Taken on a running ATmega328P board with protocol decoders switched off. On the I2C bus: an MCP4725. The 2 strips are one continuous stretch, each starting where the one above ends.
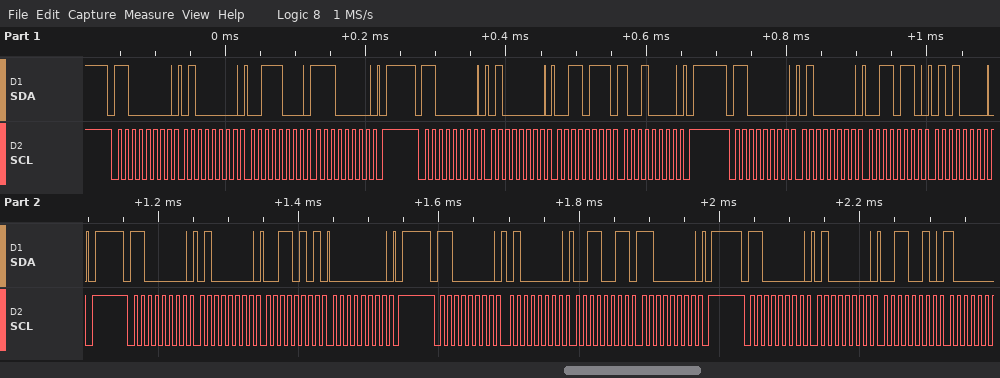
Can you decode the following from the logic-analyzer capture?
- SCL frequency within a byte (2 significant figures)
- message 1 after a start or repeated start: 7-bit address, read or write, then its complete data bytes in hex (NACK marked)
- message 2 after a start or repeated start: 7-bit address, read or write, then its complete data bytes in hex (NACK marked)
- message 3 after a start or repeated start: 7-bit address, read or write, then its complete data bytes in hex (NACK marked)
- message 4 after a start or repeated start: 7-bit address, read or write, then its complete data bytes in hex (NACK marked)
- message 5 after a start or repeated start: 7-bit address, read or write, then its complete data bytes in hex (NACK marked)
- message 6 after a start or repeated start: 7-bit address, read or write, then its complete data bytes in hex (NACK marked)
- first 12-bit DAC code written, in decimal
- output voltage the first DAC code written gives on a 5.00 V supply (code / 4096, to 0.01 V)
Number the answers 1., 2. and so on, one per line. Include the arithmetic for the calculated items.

1. 100 kHz
2. 0x60 write: 40 38 E0
3. 0x60 write: 40 37 90
4. 0x60 write: 40 36 50
5. 0x60 write: 40 35 00
6. 0x60 write: 40 33 C0
7. 0x60 write: 40 32
8. 910
9. 910 / 4096 x 5.00 V = 1.11 V
